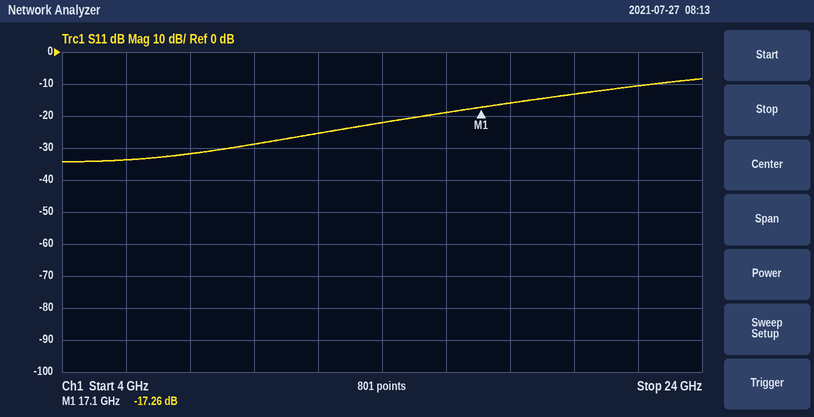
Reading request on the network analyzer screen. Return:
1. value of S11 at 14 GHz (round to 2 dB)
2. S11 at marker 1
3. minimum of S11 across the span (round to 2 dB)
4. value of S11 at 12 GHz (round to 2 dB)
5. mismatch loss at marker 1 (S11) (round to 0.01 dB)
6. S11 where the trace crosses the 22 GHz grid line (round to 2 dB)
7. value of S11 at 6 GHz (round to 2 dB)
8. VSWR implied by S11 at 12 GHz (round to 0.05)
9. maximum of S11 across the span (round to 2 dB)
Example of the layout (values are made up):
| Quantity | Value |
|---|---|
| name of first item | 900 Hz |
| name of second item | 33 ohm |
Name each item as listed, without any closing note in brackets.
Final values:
| Quantity | Value |
|---|---|
| value of S11 at 14 GHz | -22 dB |
| S11 at marker 1 | -17.26 dB |
| minimum of S11 across the span | -34 dB |
| value of S11 at 12 GHz | -26 dB |
| mismatch loss at marker 1 (S11) | 0.08 dB |
| S11 where the trace crosses the 22 GHz grid line | -10 dB |
| value of S11 at 6 GHz | -34 dB |
| VSWR implied by S11 at 12 GHz | 1.10 |
| maximum of S11 across the span | -8 dB |
